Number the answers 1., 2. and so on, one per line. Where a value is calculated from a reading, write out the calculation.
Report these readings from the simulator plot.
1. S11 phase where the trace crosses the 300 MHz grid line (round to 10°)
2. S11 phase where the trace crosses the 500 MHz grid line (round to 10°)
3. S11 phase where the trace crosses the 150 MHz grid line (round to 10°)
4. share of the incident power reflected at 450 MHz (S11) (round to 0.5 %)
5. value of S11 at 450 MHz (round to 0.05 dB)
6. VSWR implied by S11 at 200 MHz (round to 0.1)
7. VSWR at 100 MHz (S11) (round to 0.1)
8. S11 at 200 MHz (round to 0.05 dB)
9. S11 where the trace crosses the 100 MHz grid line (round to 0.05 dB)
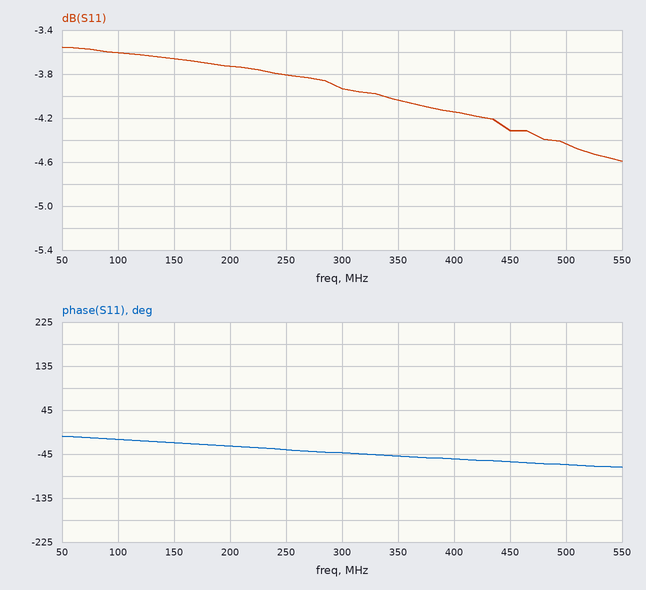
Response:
1. -40°
2. -70°
3. -20°
4. 10^(-4.3/10) ≈ 37.2 %, so 37.0 % to the nearest 0.5 %
5. -4.30 dB
6. |Γ| = 10^(-3.75/20) = 0.6494; VSWR = (1 + 0.6494)/(1 − 0.6494) ≈ 4.7
7. |Γ| = 10^(-3.6/20) = 0.6607; VSWR = (1 + 0.6607)/(1 − 0.6607) ≈ 4.9
8. -3.75 dB
9. -3.60 dB
